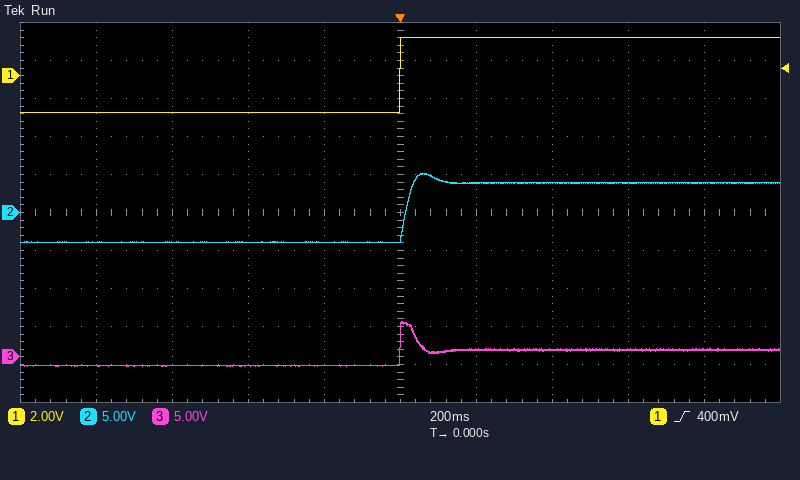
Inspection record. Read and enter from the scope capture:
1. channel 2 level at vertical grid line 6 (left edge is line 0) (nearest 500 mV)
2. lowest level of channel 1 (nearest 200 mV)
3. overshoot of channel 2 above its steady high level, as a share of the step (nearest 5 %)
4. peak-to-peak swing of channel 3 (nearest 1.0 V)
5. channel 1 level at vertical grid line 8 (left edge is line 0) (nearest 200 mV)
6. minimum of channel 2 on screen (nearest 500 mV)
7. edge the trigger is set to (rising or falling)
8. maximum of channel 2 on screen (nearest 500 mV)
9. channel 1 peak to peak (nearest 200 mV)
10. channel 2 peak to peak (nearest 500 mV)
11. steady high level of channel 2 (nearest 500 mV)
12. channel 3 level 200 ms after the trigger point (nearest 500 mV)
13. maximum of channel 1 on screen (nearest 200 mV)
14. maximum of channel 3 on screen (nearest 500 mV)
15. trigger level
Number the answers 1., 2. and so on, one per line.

1. 4.0 V
2. -2.0 V
3. 15 %
4. 6.0 V
5. 2.0 V
6. -4.0 V
7. rising
8. 5.0 V
9. 4.0 V
10. 9.0 V
11. 4.0 V
12. 1.0 V
13. 2.0 V
14. 4.5 V
15. 400 mV
